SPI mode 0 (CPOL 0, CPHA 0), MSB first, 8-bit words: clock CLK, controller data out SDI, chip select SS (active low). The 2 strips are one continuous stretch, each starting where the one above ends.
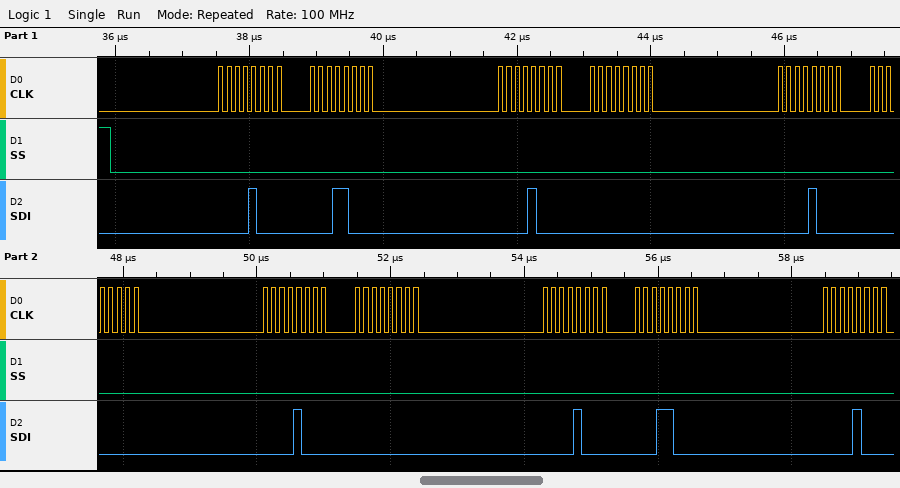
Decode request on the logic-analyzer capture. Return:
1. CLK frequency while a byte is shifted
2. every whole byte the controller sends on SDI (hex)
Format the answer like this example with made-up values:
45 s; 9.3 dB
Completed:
8 MHz; 08 18 08 00 08 00 08 00 08 18 08
